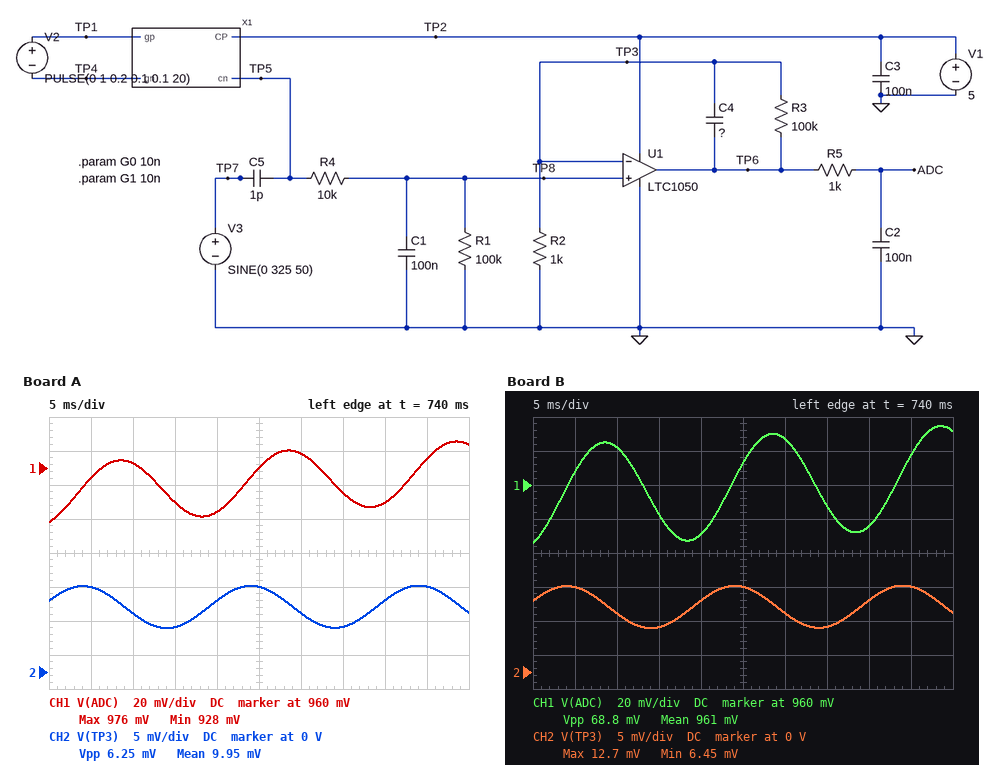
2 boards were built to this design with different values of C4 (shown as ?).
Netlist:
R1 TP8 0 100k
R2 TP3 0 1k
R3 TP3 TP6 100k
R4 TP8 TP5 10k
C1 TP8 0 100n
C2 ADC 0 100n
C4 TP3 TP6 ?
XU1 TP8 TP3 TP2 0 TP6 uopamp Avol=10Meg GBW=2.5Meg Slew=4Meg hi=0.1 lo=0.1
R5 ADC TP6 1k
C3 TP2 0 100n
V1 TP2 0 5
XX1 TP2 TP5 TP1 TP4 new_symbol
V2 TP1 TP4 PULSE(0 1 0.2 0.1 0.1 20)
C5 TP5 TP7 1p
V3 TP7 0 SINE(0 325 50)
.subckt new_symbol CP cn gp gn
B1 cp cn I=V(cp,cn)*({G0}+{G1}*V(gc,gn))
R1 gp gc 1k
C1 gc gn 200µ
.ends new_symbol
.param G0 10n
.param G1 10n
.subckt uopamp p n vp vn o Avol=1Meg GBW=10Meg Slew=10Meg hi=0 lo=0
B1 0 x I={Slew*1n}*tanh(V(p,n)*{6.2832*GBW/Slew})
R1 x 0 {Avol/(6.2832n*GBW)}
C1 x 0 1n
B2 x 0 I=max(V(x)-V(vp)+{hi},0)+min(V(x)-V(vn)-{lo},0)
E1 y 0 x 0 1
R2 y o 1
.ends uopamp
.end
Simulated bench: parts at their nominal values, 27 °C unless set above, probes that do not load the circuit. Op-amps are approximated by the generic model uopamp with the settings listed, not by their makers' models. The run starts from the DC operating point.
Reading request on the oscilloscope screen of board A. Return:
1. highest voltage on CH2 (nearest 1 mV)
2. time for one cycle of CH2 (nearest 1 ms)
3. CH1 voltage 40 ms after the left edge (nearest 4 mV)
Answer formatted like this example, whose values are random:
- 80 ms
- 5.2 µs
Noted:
- 13 mV
- 20 ms
- 940 mV
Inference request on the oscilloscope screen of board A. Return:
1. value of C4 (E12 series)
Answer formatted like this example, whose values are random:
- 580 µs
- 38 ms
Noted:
- 560 nF
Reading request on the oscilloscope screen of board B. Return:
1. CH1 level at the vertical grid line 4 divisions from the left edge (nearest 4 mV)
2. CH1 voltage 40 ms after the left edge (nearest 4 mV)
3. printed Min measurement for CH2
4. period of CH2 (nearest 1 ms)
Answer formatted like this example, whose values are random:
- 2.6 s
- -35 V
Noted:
- 932 mV
- 936 mV
- 6.45 mV
- 20 ms
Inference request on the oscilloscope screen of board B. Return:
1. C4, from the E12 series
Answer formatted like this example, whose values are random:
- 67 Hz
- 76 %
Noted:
- 330 nF
